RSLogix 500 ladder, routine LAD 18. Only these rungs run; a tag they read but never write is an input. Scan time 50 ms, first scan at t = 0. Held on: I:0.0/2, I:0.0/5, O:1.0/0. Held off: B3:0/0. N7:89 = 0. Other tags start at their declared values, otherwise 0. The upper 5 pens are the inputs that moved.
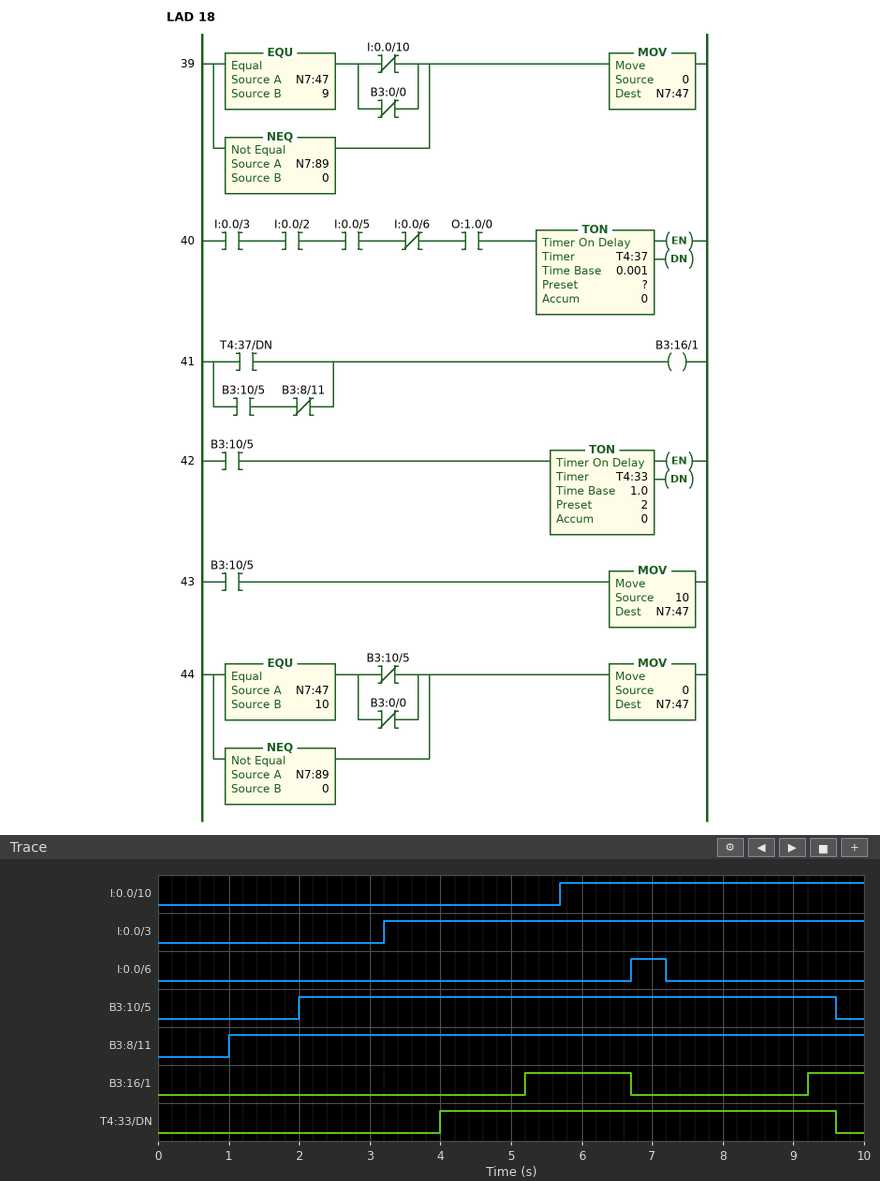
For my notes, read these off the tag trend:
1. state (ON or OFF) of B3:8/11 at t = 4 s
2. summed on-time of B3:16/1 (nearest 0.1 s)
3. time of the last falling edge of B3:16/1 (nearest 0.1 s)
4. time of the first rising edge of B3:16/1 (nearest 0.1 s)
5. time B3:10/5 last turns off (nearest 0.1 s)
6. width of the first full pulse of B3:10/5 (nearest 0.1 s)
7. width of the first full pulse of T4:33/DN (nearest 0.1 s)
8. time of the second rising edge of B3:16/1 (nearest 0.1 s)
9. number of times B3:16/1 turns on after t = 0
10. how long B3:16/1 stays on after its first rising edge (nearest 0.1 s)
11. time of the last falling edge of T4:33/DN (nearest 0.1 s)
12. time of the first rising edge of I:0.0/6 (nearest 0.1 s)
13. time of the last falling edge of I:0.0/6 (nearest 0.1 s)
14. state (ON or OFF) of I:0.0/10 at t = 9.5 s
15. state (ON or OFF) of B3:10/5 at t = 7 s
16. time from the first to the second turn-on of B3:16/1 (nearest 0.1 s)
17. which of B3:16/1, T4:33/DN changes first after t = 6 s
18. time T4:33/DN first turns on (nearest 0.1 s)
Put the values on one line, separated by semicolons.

ON; 2.3 s; 6.7 s; 5.2 s; 9.6 s; 7.6 s; 5.6 s; 9.2 s; 2; 1.5 s; 9.6 s; 6.7 s; 7.2 s; ON; ON; 4.0 s; B3:16/1; 4.0 s
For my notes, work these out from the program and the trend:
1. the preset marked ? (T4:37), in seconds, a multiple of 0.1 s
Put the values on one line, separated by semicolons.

2.0 s
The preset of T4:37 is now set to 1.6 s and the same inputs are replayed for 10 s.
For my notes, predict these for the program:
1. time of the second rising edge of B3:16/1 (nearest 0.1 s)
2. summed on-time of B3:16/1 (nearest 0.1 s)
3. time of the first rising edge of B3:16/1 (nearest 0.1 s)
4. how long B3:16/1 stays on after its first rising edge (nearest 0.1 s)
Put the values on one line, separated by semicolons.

8.8 s; 3.1 s; 4.8 s; 1.9 s
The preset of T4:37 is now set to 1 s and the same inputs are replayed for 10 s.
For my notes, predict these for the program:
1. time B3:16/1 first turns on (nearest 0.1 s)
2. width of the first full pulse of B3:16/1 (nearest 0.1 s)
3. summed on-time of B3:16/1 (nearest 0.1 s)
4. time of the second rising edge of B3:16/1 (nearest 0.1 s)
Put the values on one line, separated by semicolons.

4.2 s; 2.5 s; 4.3 s; 8.2 s
